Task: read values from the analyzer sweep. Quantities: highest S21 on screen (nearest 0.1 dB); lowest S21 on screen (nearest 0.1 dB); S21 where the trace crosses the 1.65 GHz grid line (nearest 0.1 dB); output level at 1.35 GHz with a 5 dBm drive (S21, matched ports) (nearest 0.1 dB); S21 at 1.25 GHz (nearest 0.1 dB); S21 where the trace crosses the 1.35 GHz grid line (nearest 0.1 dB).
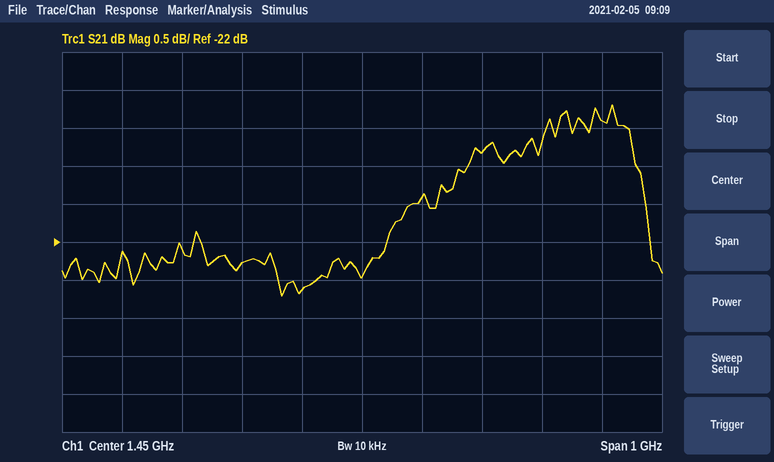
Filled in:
-20.2 dB
-22.7 dB
-20.8 dB
-17.6 dBm
-22.3 dB
-22.6 dB
